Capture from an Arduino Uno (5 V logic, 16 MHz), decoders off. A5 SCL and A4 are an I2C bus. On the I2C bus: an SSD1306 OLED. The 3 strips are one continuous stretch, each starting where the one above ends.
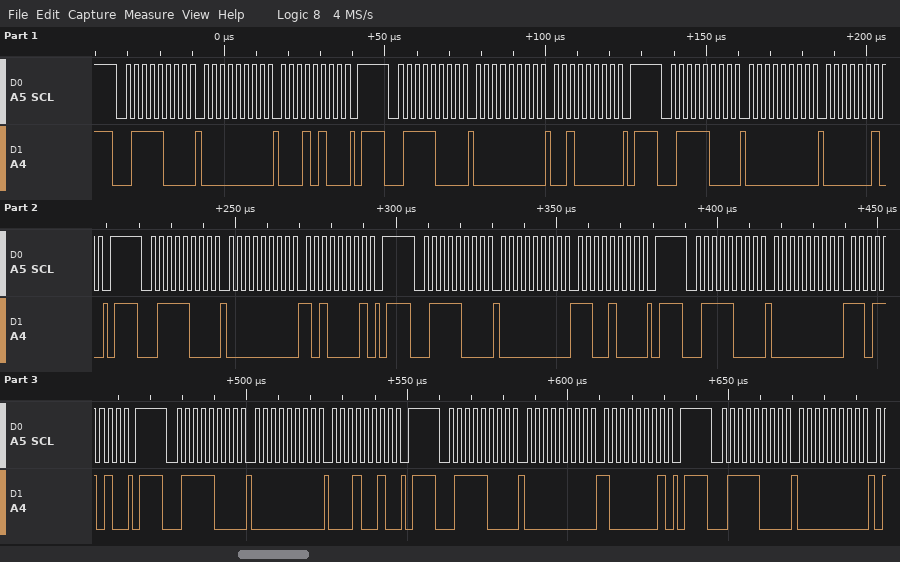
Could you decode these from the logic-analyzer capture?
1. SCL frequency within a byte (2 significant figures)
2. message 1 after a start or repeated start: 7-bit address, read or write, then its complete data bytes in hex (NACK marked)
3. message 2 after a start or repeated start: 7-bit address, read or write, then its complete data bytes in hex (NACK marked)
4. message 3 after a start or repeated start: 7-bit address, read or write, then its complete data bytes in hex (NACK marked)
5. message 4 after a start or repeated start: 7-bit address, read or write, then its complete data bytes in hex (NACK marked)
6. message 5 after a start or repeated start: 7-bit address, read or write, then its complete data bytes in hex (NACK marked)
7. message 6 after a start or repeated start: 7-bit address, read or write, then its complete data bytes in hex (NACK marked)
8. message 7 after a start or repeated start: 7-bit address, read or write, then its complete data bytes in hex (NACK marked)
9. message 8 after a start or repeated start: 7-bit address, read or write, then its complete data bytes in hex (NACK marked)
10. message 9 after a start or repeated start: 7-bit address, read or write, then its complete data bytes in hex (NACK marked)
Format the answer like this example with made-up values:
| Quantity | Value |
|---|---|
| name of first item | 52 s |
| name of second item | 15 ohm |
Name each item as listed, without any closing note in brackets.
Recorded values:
| Quantity | Value |
|---|---|
| SCL frequency within a byte | 400 kHz |
| message 1 after a start or repeated start: 7-bit address, read or write, then its complete data bytes in hex | 0x3C write: 00 14 |
| message 2 after a start or repeated start: 7-bit address, read or write, then its complete data bytes in hex | 0x3C write: 00 20 |
| message 3 after a start or repeated start: 7-bit address, read or write, then its complete data bytes in hex | 0x3C write: 00 02 |
| message 4 after a start or repeated start: 7-bit address, read or write, then its complete data bytes in hex | 0x3C write: 00 A1 |
| message 5 after a start or repeated start: 7-bit address, read or write, then its complete data bytes in hex | 0x3C write: 00 C8 |
| message 6 after a start or repeated start: 7-bit address, read or write, then its complete data bytes in hex | 0x3C write: 00 DA |
| message 7 after a start or repeated start: 7-bit address, read or write, then its complete data bytes in hex | 0x3C write: 00 12 |
| message 8 after a start or repeated start: 7-bit address, read or write, then its complete data bytes in hex | 0x3C write: 00 81 |
| message 9 after a start or repeated start: 7-bit address, read or write, then its complete data bytes in hex | 0x3C write: 00 |
